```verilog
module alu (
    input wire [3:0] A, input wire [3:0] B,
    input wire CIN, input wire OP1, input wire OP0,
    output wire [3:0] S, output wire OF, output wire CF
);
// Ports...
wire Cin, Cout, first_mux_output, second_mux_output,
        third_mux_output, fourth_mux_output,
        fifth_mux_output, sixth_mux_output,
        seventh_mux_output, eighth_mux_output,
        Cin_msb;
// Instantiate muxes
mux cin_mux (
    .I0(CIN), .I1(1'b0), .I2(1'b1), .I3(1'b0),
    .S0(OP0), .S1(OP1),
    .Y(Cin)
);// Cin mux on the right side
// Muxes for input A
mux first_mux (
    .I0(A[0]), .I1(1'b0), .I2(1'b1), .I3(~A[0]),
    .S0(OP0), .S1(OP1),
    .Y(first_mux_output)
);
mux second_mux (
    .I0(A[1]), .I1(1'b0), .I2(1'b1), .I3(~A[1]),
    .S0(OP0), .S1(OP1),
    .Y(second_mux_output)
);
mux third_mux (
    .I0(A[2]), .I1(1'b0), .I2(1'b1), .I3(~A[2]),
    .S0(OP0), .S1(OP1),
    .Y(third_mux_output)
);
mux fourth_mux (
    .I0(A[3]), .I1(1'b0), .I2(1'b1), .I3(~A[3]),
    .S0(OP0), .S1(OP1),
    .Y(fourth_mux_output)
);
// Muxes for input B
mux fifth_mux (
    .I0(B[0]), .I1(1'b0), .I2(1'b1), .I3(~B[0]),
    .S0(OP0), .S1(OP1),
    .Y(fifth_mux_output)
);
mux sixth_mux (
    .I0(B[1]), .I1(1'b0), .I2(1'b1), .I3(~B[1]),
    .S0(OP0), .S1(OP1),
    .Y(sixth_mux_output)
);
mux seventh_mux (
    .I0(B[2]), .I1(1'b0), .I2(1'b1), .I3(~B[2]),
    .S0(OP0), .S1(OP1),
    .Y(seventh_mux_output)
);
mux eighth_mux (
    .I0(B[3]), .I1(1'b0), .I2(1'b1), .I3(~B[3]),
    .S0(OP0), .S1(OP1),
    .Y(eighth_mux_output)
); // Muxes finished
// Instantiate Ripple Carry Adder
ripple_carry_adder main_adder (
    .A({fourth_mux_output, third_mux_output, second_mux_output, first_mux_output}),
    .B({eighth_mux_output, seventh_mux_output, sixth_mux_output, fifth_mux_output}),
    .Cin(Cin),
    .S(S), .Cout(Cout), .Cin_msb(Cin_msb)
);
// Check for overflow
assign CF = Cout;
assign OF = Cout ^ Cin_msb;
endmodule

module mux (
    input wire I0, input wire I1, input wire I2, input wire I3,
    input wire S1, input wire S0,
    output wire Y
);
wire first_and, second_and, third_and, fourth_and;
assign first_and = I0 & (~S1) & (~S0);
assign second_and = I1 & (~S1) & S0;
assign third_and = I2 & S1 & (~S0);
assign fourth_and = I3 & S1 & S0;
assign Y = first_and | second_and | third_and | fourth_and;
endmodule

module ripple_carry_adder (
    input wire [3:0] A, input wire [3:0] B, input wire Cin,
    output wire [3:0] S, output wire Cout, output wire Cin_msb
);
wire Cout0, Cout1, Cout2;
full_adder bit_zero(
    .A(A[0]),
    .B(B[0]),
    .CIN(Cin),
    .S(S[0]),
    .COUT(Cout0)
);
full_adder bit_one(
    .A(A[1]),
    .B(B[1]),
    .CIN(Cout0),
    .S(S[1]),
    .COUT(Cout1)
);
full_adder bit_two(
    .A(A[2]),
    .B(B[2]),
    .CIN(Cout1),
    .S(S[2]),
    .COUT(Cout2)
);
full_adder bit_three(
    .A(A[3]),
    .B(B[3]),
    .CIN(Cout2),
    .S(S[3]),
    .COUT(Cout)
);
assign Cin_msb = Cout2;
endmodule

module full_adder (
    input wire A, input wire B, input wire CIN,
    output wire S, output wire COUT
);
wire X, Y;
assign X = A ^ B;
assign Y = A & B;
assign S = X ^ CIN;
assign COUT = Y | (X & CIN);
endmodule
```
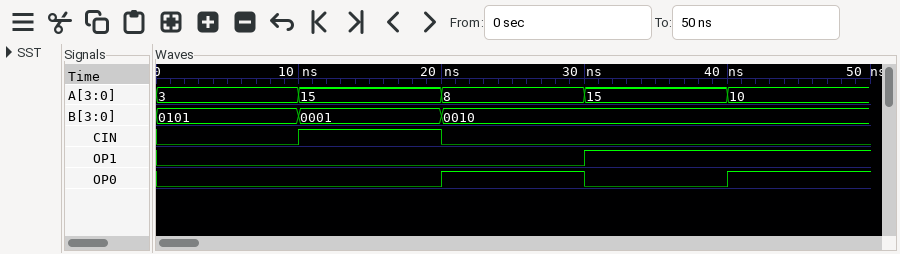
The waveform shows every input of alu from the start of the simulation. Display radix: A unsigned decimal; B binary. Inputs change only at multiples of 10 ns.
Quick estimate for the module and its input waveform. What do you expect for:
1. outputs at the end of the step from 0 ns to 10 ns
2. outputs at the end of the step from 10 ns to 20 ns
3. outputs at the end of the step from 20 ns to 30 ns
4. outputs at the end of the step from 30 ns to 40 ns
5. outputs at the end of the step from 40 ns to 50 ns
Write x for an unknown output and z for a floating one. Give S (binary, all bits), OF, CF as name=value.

S=1000, OF=1, CF=0
S=0001, OF=0, CF=1
S=0000, OF=0, CF=0
S=1111, OF=0, CF=1
S=0010, OF=0, CF=1
